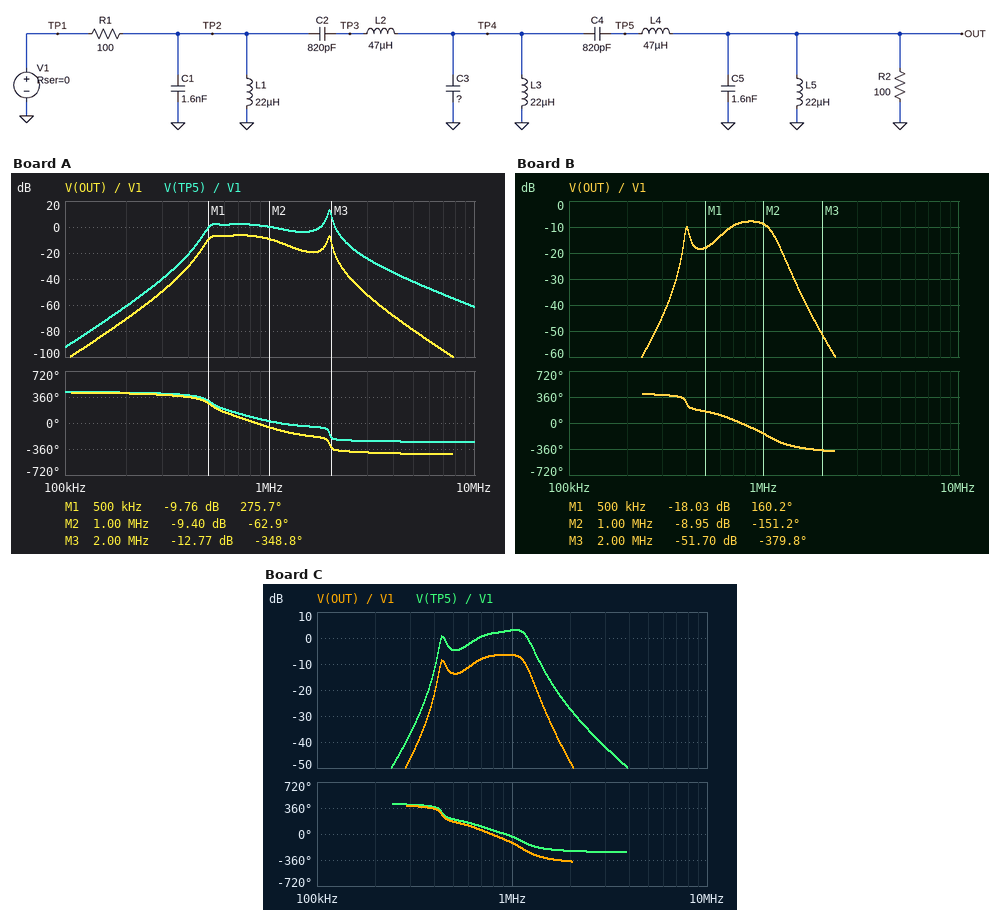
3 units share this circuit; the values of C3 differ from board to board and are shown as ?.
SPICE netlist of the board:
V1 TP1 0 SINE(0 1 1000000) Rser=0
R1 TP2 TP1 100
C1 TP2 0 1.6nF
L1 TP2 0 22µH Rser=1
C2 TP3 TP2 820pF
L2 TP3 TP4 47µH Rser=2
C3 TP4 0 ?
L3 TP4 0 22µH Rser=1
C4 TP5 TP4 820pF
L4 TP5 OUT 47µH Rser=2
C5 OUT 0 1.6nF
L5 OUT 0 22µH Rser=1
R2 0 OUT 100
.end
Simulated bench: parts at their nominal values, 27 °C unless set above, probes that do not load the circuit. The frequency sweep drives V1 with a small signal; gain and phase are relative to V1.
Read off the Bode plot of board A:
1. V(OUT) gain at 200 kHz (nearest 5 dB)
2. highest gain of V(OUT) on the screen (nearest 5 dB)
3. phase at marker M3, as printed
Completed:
-70 dB
-5 dB
-348.8 deg
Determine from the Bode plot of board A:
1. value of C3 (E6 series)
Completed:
680 pF
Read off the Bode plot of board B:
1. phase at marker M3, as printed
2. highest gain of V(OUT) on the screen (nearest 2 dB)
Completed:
-379.8 deg
-8 dB
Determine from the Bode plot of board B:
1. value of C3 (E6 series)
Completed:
4.7 nF
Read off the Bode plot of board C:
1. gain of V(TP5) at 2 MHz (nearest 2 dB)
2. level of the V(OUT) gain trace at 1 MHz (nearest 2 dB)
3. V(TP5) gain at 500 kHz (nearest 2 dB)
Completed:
-28 dB
-6 dB
-4 dB
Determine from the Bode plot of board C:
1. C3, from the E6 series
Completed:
3.3 nF
